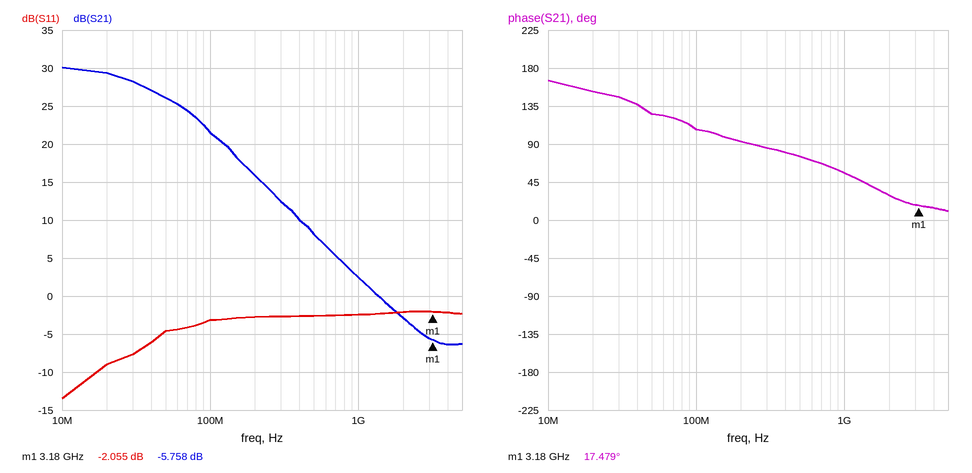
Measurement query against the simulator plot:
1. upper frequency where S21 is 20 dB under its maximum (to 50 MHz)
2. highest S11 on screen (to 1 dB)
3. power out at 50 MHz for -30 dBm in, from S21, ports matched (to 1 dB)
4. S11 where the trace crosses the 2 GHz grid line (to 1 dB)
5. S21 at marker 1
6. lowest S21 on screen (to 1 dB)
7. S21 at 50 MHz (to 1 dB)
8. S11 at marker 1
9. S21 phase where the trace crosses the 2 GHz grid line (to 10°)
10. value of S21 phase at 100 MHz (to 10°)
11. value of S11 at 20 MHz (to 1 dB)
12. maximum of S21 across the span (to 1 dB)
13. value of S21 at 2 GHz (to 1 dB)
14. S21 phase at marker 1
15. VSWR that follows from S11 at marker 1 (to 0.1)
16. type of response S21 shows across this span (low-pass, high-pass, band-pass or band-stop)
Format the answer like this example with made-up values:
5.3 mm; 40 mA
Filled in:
400 MHz; -2 dB; -4 dBm; -2 dB; -5.758 dB; -6 dB; 26 dB; -2.055 dB; 30°; 110°; -9 dB; 30 dB; -3 dB; 17.479°; 8.5; low-pass
